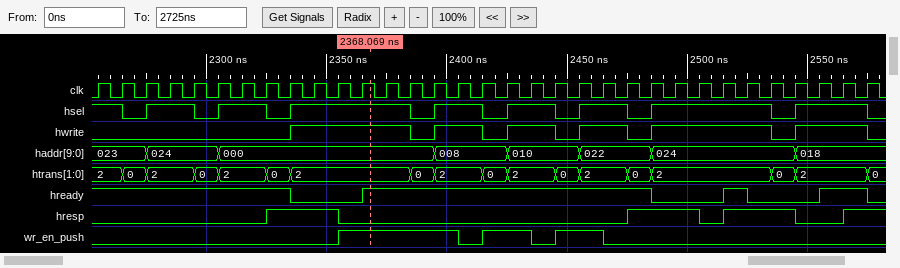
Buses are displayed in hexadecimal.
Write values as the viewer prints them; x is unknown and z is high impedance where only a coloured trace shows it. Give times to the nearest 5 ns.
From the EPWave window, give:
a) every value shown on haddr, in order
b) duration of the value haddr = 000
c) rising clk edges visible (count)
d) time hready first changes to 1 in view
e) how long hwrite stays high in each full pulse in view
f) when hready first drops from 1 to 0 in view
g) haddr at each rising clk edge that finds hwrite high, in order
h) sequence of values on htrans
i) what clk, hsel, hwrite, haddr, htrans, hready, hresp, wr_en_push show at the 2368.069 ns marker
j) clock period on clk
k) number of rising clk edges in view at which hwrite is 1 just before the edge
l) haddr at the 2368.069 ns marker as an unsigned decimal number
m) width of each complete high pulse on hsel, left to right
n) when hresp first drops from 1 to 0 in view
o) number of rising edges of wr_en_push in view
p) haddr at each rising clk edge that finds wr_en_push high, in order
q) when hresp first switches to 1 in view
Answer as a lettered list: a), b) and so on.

a) 023, 024, 000, 008, 010, 022, 024, 018
b) 90 ns
c) 33
d) 2365 ns
e) 50 ns, 20 ns, 20 ns, 20 ns, 50 ns, 30 ns
f) 2335 ns
g) 000, 000, 000, 000, 000, 008, 008, 010, 010, 022, 022, 024, 024, 024, 024, 024, 018, 018, 018
h) 2, 0, 2, 0, 2, 0, 2, 0, 2, 0, 2, 0, 2, 0, 2, 0, 2, 0
i) clk=1, hsel=1, hwrite=1, haddr=000, htrans=2, hready=1, hresp=0, wr_en_push=1
j) 10 ns
k) 19
l) 0
m) 20 ns, 20 ns, 50 ns, 20 ns, 20 ns, 20 ns, 50 ns, 30 ns
n) 2355 ns
o) 3
p) 000, 000, 000, 000, 008, 008, 010, 010, 022
q) 2325 ns
